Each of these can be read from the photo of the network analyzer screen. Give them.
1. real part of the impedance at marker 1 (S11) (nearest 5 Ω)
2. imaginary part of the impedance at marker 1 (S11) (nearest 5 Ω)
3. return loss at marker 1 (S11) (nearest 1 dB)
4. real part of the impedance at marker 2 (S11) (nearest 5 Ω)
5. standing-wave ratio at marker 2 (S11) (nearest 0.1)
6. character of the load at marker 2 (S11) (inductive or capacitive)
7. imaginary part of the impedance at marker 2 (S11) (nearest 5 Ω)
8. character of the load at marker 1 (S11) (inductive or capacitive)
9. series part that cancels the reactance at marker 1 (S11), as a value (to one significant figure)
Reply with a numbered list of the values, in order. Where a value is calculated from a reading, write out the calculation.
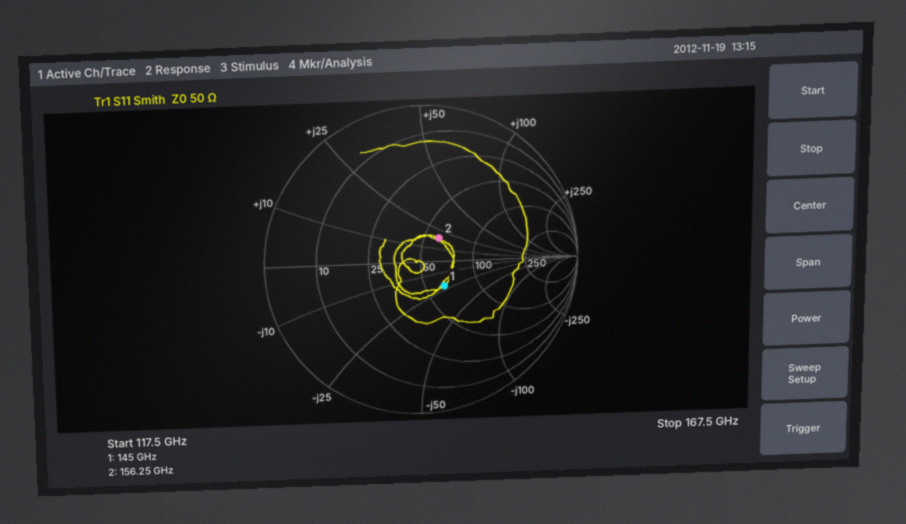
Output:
1. 65 Ω
2. -20 Ω
3. 13 dB
4. 60 Ω
5. 1.5
6. inductive
7. +20 Ω
8. capacitive
9. L = 20 Ω/(2π × 145 GHz) ≈ 22.0 pH, so 20 pH to one significant figure
